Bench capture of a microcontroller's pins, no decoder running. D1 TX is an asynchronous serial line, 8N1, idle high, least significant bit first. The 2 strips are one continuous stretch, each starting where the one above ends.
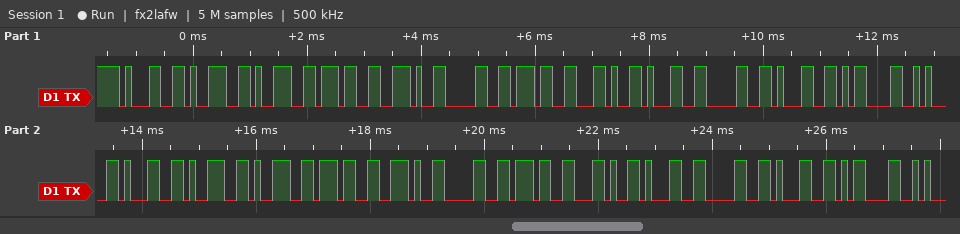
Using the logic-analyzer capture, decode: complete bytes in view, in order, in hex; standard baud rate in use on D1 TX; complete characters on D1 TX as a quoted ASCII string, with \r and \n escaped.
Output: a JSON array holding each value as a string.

["31 39 39 37 2E 30 37 2C 31 30 31 0D 0A 31 39 39 37 2E 30 37 2C 31 30 31 0D", "9600 baud", "\"1997.07,101\\r\\n1997.07,101\\r\""]
